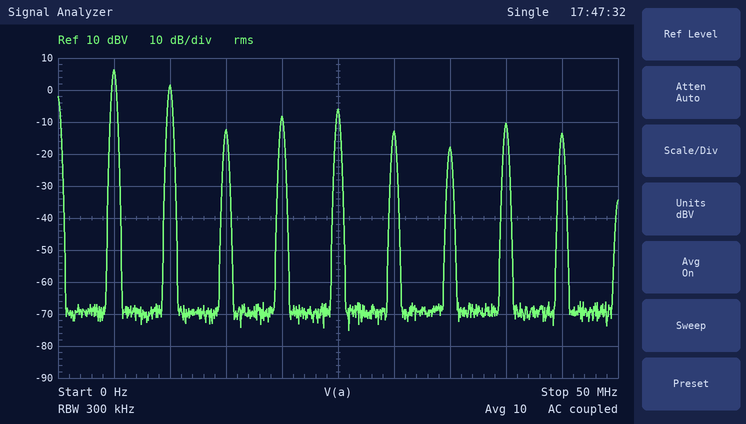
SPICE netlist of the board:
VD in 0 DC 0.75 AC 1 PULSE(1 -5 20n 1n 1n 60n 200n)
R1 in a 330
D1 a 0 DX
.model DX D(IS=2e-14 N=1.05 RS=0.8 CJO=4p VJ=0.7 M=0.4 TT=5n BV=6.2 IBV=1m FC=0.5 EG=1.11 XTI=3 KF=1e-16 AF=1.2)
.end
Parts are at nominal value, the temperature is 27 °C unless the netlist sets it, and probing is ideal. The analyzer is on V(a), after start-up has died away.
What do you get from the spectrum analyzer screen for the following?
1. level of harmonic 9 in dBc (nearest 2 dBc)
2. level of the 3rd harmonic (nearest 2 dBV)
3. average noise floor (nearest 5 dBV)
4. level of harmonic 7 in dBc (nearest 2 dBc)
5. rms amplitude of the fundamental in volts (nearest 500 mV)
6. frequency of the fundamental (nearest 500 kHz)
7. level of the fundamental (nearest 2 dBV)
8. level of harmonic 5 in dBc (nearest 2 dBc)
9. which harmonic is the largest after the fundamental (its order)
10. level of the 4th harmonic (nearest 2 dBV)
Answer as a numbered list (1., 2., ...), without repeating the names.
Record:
1. -20 dBc
2. -12 dBV
3. -70 dBV
4. -24 dBc
5. 2.0 V
6. 5.0 MHz
7. 6 dBV
8. -12 dBc
9. 2
10. -8 dBV
